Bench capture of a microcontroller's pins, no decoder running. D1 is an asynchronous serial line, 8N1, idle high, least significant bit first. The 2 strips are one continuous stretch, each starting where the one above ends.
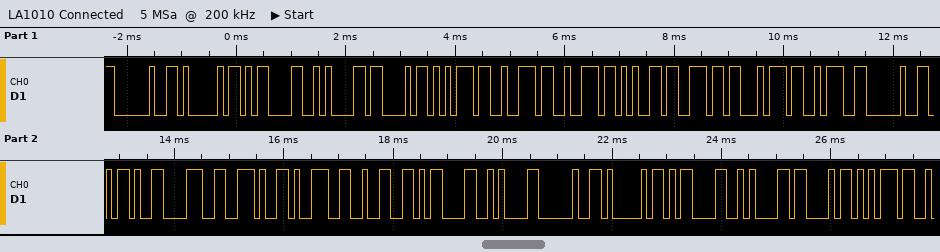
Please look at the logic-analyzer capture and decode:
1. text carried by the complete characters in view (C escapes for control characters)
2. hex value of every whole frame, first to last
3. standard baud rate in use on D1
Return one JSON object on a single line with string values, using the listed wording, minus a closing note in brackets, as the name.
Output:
{"text carried by the complete characters in view": "\" A\\r\\nCurrent: -8.92\\r\\n A\\r\\nCu\"", "hex value of every whole frame, first to last": "0x20 0x41 0x0D 0x0A 0x43 0x75 0x72 0x72 0x65 0x6E 0x74 0x3A 0x20 0x2D 0x38 0x2E 0x39 0x32 0x0D 0x0A 0x20 0x41 0x0D 0x0A 0x43 0x75", "standard baud rate in use on D1": "9600 baud"}
